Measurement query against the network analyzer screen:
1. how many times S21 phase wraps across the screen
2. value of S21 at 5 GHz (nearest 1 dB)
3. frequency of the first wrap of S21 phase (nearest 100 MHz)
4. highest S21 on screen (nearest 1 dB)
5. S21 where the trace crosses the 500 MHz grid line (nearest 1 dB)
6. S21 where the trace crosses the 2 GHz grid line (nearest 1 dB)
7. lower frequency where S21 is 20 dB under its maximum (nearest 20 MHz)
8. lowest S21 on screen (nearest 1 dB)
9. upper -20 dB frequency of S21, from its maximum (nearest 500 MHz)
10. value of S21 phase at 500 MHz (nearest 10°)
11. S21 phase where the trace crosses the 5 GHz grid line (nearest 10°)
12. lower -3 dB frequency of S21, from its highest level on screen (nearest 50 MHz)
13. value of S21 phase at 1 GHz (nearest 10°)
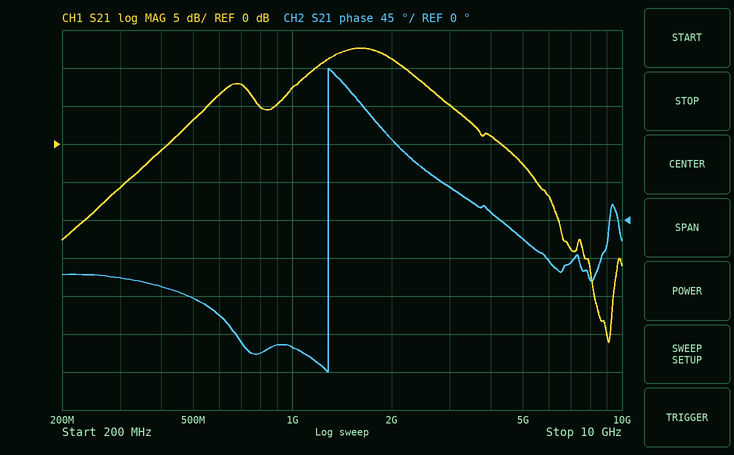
1
-3 dB
1.3 GHz
13 dB
3 dB
11 dB
280 MHz
-26 dB
6.0 GHz
-90°
-20°
1.15 GHz
-150°
